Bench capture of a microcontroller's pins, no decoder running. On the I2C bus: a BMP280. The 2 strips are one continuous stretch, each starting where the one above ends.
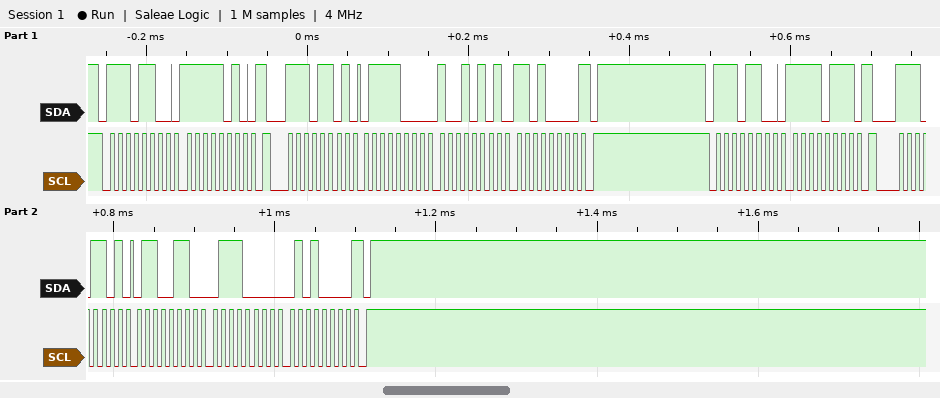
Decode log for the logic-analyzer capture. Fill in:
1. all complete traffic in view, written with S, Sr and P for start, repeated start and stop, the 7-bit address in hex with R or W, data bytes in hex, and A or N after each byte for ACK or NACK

S 76W A FA A Sr 76R A 78 A 95 A D0 N P S 76W A F7 A Sr 76R A 66 A 70 A 50 N P
